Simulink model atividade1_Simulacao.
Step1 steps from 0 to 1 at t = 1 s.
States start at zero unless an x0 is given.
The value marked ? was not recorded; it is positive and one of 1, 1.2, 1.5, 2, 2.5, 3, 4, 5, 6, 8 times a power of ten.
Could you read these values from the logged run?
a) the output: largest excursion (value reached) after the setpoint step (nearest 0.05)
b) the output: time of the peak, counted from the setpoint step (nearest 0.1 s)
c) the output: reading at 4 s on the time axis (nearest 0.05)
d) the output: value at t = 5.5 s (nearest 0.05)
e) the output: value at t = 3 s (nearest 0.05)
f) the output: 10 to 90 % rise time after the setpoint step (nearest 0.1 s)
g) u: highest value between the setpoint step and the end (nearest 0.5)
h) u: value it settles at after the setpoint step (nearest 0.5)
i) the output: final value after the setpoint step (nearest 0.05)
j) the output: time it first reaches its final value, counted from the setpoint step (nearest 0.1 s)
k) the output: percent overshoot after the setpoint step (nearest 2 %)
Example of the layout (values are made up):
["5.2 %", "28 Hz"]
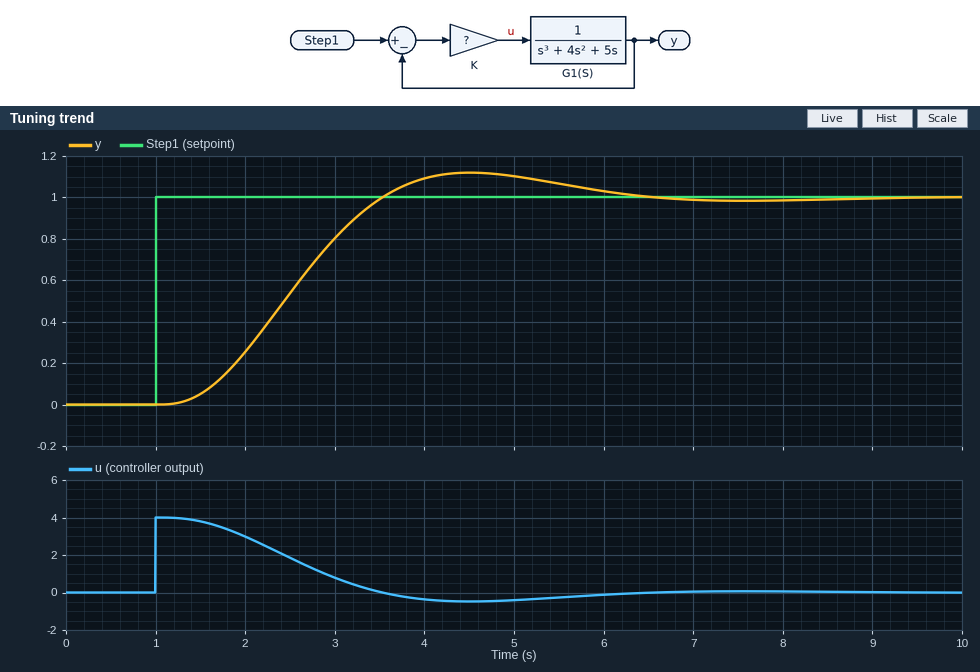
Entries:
["1.10", "3.5 s", "1.10", "1.05", "0.80", "1.6 s", "4.0", "0.0", "1.00", "2.5 s", "12 %"]
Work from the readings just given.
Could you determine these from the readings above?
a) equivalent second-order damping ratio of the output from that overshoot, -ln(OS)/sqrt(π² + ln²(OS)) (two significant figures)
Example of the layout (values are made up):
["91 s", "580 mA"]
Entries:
["0.56"]
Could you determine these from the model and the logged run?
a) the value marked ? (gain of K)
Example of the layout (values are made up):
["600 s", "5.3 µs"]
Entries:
["4"]
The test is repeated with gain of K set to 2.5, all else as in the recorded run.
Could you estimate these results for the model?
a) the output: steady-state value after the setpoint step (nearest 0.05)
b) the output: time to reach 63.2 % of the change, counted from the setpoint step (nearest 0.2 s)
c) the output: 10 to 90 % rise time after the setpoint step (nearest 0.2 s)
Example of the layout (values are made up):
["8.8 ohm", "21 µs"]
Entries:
["1.00", "2.2 s", "2.6 s"]
